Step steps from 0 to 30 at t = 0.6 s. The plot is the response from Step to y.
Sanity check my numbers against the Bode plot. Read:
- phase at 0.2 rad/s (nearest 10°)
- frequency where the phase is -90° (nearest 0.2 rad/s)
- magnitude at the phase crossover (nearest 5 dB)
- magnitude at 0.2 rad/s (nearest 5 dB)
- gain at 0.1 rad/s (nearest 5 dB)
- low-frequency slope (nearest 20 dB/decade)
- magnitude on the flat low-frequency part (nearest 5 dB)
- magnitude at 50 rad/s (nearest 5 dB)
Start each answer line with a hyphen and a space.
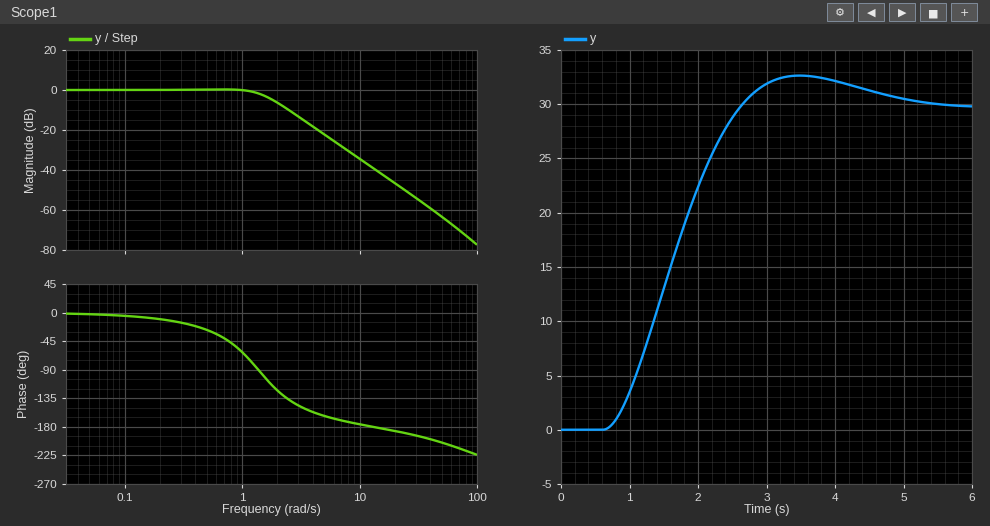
- -10°
- 1.4 rad/s
- -40 dB
- 0 dB
- 0 dB
- 0 dB/decade
- 0 dB
- -65 dB
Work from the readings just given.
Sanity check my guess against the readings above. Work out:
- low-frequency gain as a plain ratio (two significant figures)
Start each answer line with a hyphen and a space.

- 1.0
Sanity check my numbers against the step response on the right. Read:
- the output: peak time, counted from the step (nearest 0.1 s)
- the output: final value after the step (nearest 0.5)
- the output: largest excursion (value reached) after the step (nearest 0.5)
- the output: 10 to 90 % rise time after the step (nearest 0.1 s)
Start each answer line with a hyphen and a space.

- 2.9 s
- 30.0
- 32.5
- 1.4 s
